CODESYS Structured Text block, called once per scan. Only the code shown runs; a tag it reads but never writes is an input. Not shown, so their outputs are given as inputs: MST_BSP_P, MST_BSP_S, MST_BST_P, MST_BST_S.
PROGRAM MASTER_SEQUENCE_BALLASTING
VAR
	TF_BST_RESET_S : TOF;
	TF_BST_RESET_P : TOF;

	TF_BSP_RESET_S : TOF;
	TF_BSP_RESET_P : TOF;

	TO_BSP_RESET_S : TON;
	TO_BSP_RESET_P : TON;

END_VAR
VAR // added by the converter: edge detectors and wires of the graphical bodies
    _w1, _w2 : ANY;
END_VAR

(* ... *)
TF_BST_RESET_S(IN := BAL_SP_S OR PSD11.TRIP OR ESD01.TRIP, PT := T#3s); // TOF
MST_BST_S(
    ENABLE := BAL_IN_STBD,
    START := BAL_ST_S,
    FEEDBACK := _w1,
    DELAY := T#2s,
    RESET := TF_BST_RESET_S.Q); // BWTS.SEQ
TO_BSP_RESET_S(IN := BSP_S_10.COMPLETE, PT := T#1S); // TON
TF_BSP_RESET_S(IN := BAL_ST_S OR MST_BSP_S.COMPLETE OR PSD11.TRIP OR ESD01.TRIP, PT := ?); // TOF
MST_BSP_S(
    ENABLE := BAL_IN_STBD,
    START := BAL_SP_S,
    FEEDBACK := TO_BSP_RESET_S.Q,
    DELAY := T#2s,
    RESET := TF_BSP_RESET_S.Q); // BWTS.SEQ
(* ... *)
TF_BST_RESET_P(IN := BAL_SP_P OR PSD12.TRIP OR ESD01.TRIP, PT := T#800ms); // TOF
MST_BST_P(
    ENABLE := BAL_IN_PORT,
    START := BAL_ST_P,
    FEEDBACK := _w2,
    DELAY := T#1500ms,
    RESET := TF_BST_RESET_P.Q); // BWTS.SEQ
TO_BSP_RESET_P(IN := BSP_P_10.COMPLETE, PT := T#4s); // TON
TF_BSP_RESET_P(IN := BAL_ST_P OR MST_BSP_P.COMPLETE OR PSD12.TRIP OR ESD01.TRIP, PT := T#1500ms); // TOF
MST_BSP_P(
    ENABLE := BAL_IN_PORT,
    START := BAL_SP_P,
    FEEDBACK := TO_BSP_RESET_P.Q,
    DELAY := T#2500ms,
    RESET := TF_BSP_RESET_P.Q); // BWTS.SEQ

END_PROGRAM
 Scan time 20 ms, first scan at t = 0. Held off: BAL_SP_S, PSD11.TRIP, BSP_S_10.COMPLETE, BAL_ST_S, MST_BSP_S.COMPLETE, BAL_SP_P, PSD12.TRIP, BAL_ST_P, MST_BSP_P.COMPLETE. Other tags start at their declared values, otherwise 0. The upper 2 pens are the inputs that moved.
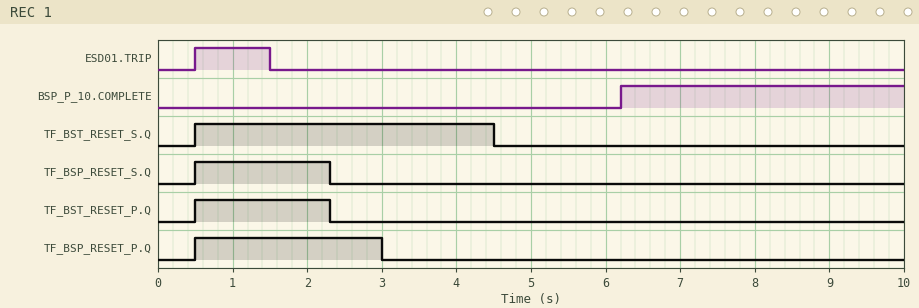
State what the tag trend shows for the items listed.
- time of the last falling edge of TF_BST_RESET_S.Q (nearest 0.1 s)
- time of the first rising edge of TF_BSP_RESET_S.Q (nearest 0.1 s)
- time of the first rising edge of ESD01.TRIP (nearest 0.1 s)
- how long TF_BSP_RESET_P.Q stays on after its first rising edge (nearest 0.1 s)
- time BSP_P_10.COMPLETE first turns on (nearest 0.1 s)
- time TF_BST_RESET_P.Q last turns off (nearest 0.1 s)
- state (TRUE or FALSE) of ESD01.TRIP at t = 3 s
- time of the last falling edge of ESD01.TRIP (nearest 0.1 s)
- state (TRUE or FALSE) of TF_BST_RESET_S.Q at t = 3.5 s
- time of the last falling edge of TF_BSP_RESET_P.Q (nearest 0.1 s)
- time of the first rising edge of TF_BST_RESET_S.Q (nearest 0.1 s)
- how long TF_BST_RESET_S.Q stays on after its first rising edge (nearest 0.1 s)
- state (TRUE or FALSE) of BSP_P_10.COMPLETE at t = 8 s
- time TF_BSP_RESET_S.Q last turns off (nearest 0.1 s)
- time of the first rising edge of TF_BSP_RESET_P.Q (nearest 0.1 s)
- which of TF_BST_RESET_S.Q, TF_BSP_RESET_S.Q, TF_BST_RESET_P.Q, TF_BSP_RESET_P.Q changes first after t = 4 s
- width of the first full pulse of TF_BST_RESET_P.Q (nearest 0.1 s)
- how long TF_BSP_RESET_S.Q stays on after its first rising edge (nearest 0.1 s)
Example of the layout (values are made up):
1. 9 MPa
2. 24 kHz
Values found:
1. 4.5 s
2. 0.5 s
3. 0.5 s
4. 2.5 s
5. 6.2 s
6. 2.3 s
7. FALSE
8. 1.5 s
9. TRUE
10. 3.0 s
11. 0.5 s
12. 4.0 s
13. TRUE
14. 2.3 s
15. 0.5 s
16. TF_BST_RESET_S.Q
17. 1.8 s
18. 1.8 s
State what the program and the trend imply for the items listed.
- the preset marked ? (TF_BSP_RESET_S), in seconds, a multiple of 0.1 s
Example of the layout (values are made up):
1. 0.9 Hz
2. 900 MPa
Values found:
1. 0.8 s
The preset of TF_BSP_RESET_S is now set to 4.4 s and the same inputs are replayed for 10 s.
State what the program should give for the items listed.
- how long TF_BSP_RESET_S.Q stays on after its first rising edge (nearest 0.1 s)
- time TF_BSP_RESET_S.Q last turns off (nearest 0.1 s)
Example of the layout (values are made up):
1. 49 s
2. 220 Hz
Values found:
1. 5.4 s
2. 5.9 s
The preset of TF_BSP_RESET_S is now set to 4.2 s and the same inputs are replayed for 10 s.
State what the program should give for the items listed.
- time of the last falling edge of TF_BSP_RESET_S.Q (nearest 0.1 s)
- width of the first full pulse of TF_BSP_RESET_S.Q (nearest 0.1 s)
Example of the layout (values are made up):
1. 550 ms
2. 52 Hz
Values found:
1. 5.7 s
2. 5.2 s
